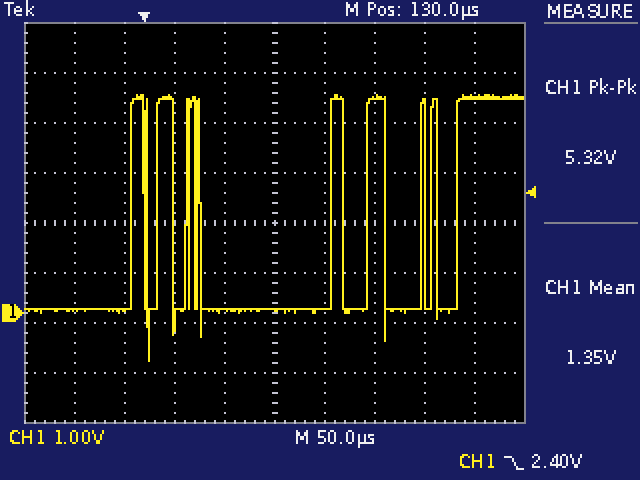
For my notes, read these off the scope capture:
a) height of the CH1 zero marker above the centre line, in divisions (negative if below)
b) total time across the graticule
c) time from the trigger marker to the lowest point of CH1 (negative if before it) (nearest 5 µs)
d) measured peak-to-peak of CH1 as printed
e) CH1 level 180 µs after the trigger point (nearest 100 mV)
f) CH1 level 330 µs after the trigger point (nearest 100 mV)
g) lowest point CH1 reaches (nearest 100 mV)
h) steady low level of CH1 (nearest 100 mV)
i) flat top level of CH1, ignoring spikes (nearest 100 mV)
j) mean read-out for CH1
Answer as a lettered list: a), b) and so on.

a) -1.8 div
b) 500 µs
c) +5 µs
d) 5.32 V
e) 100 mV
f) 4.3 V
g) -1.0 V
h) 100 mV
i) 4.3 V
j) 1.35 V
